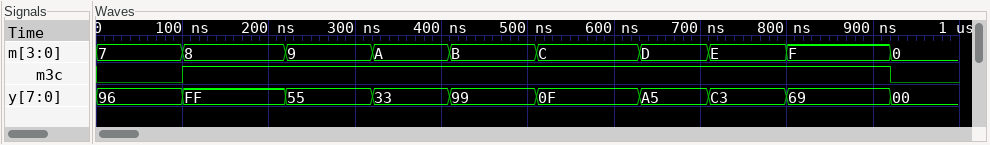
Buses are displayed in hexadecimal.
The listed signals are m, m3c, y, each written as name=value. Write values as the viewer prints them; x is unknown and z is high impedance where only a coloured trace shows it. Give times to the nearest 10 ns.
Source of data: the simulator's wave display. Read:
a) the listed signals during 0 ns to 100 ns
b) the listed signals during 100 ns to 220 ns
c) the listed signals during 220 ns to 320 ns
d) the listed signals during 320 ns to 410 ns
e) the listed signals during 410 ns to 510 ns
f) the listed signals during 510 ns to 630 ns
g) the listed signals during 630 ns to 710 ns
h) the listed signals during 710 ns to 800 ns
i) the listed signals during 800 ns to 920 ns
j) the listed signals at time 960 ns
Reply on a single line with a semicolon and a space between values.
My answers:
m=7, m3c=0, y=96; m=8, m3c=1, y=FF; m=9, m3c=1, y=55; m=A, m3c=1, y=33; m=B, m3c=1, y=99; m=C, m3c=1, y=0F; m=D, m3c=1, y=A5; m=E, m3c=1, y=C3; m=F, m3c=1, y=69; m=0, m3c=0, y=00
